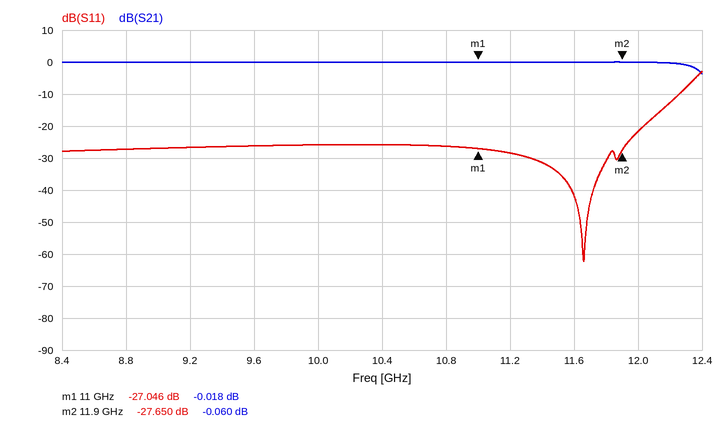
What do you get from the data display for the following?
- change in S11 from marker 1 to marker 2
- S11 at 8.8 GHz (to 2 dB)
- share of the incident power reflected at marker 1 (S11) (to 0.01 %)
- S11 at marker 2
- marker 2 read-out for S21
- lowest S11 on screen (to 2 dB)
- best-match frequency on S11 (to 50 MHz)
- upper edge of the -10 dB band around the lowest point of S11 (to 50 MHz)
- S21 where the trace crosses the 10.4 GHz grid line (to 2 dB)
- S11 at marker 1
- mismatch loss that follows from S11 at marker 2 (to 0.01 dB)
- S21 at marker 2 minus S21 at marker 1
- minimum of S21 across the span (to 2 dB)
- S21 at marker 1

-0.604 dB
-28 dB
0.20 %
-27.650 dB
-0.060 dB
-62 dB
11.65 GHz
12.25 GHz
0 dB
-27.046 dB
0.01 dB
-0.042 dB
-4 dB
-0.018 dB
